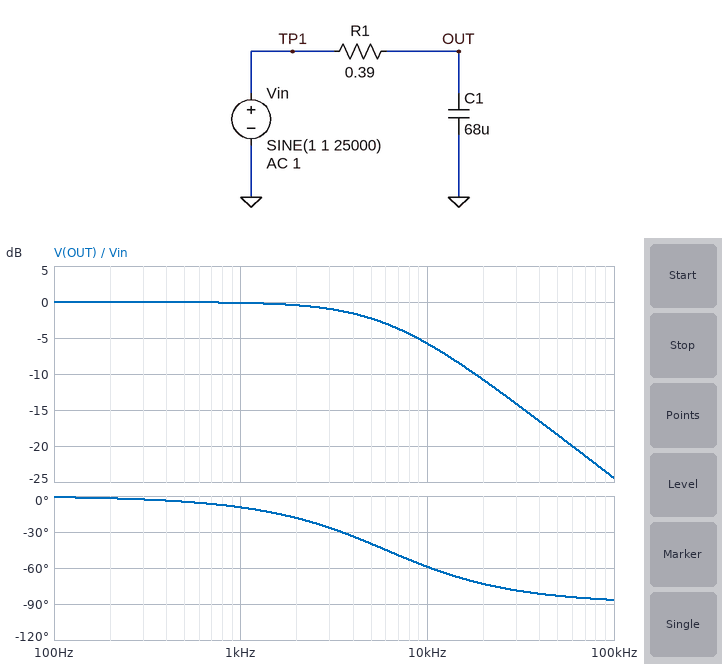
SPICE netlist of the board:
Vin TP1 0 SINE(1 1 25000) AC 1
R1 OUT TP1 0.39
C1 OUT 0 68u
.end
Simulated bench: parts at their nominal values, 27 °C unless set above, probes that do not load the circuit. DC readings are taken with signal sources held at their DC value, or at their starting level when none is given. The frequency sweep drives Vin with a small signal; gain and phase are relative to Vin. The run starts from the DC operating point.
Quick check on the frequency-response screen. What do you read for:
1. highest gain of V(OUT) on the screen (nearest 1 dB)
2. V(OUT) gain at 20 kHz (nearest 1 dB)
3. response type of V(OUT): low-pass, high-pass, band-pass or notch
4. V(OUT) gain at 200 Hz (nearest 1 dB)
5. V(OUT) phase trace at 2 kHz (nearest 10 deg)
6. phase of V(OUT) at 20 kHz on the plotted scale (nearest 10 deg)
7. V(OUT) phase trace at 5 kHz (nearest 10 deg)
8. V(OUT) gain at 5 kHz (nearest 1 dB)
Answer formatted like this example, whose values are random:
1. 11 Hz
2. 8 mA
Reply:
1. 0 dB
2. -11 dB
3. low-pass
4. 0 dB
5. -20 deg
6. -70 deg
7. -40 deg
8. -2 dB
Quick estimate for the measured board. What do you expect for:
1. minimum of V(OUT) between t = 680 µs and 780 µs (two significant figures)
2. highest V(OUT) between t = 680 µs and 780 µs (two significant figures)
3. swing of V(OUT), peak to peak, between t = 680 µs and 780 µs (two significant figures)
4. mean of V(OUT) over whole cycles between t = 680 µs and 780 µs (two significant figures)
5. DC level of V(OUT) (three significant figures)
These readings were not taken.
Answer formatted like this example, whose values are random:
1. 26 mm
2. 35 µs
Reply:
1. 770 mV
2. 1.2 V
3. 470 mV
4. 1.0 V
5. 1.00 V
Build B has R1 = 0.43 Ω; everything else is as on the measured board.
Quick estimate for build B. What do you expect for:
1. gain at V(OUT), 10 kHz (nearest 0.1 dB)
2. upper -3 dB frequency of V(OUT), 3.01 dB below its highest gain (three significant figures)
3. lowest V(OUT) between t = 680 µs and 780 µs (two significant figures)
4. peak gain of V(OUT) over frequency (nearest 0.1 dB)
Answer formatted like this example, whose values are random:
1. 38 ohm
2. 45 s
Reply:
1. -6.4 dB
2. 5.44 kHz
3. 790 mV
4. 0 dB
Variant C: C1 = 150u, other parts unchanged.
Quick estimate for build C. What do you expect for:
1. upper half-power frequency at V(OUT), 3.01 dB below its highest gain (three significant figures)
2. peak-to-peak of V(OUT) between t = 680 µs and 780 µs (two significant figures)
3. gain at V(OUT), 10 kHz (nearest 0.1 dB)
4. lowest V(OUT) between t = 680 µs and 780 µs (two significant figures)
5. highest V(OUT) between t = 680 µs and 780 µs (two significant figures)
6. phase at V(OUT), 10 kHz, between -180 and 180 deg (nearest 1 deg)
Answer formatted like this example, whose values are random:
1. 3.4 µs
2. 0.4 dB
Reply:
1. 2.72 kHz
2. 220 mV
3. -11.6 dB
4. 890 mV
5. 1.1 V
6. -75 deg
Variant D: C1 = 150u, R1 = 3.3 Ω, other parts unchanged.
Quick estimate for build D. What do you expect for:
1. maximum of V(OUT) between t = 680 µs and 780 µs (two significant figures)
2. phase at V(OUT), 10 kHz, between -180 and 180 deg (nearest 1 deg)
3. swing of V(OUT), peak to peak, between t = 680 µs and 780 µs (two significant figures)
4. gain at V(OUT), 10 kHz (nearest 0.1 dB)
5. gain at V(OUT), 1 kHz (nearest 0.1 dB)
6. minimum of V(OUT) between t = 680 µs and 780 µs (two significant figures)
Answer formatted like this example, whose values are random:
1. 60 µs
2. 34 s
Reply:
1. 1.0 V
2. -88 deg
3. 26 mV
4. -29.9 dB
5. -10.3 dB
6. 990 mV
